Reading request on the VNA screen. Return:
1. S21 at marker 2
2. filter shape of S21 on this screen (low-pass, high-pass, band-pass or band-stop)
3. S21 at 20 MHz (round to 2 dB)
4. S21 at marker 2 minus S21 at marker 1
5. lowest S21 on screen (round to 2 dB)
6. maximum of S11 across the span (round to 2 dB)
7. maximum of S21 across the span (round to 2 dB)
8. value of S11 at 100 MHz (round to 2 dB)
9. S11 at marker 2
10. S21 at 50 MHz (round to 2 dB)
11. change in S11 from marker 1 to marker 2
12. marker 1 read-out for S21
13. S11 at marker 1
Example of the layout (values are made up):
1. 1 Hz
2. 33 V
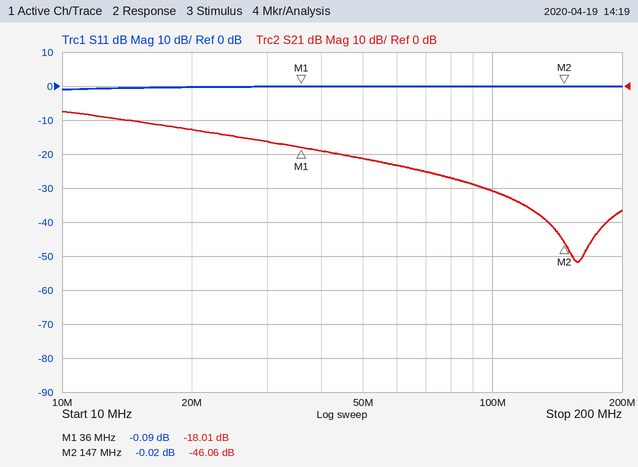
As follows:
1. -46.06 dB
2. low-pass
3. -12 dB
4. -28.05 dB
5. -52 dB
6. 0 dB
7. -8 dB
8. 0 dB
9. -0.02 dB
10. -22 dB
11. 0.07 dB
12. -18.01 dB
13. -0.09 dB
